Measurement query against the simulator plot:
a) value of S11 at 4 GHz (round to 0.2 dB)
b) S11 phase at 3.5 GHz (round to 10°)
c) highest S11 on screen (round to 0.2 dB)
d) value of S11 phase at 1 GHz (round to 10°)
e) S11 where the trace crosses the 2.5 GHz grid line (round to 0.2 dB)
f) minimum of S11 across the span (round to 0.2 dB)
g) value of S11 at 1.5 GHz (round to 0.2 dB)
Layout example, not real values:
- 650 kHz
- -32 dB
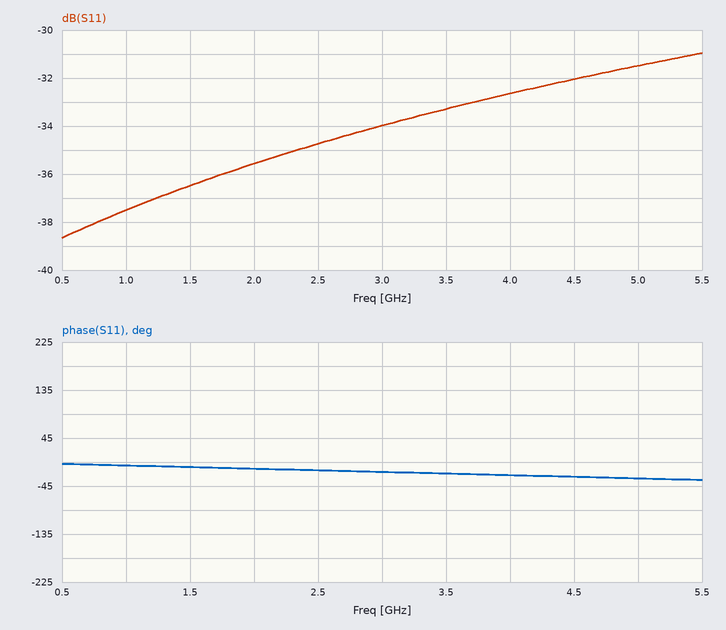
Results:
- -32.6 dB
- -20°
- -31.0 dB
- -10°
- -34.8 dB
- -38.6 dB
- -36.4 dB
